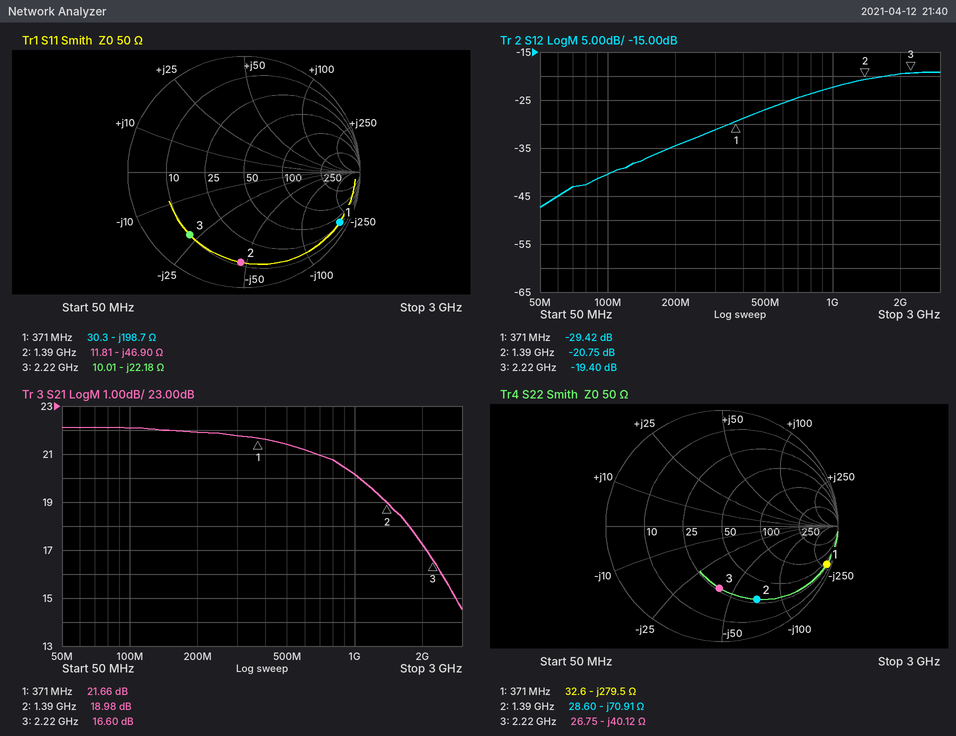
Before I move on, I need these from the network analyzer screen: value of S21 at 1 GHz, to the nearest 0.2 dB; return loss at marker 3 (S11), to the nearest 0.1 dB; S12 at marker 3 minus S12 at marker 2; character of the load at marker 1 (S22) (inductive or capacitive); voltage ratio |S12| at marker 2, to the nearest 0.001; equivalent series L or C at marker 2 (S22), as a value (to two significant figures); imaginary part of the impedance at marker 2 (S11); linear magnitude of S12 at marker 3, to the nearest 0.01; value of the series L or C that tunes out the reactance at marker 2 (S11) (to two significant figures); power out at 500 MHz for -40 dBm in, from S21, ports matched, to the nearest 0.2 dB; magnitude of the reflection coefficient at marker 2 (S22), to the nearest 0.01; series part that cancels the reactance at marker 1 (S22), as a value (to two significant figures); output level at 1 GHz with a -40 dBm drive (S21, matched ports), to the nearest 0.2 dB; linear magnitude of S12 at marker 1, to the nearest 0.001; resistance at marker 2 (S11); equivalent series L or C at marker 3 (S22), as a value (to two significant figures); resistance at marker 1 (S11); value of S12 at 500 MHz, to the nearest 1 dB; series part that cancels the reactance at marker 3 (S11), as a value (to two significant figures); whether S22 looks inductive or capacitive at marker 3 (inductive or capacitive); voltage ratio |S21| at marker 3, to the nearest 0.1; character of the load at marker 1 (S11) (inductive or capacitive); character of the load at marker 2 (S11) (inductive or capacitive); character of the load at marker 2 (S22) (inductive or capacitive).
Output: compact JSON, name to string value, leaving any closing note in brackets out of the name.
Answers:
{"value of S21 at 1 GHz, to the nearest 0.2 dB": "20.2 dB", "return loss at marker 3 (S11), to the nearest 0.1 dB": "2.9 dB", "S12 at marker 3 minus S12 at marker 2": "1.35 dB", "character of the load at marker 1 (S22)": "capacitive", "voltage ratio |S12| at marker 2, to the nearest 0.001": "0.092", "equivalent series L or C at marker 2 (S22), as a value": "1.6 pF", "imaginary part of the impedance at marker 2": "-46.90 Ω", "linear magnitude of S12 at marker 3, to the nearest 0.01": "0.11", "value of the series L or C that tunes out the reactance at marker 2 (S11)": "5.4 nH", "power out at 500 MHz for -40 dBm in, from S21, ports matched, to the nearest 0.2 dB": "-18.6 dBm", "magnitude of the reflection coefficient at marker 2 (S22), to the nearest 0.01": "0.70", "series part that cancels the reactance at marker 1 (S22), as a value": "120 nH", "output level at 1 GHz with a -40 dBm drive (S21, matched ports), to the nearest 0.2 dB": "-19.8 dBm", "linear magnitude of S12 at marker 1, to the nearest 0.001": "0.034", "resistance at marker 2": "11.81 Ω", "equivalent series L or C at marker 3 (S22), as a value": "1.8 pF", "resistance at marker 1": "30.3 Ω", "value of S12 at 500 MHz, to the nearest 1 dB": "-27 dB", "series part that cancels the reactance at marker 3 (S11), as a value": "1.6 nH", "whether S22 looks inductive or capacitive at marker 3": "capacitive", "voltage ratio |S21| at marker 3, to the nearest 0.1": "6.8", "character of the load at marker 1 (S11)": "capacitive", "character of the load at marker 2 (S11)": "capacitive", "character of the load at marker 2 (S22)": "capacitive"}
